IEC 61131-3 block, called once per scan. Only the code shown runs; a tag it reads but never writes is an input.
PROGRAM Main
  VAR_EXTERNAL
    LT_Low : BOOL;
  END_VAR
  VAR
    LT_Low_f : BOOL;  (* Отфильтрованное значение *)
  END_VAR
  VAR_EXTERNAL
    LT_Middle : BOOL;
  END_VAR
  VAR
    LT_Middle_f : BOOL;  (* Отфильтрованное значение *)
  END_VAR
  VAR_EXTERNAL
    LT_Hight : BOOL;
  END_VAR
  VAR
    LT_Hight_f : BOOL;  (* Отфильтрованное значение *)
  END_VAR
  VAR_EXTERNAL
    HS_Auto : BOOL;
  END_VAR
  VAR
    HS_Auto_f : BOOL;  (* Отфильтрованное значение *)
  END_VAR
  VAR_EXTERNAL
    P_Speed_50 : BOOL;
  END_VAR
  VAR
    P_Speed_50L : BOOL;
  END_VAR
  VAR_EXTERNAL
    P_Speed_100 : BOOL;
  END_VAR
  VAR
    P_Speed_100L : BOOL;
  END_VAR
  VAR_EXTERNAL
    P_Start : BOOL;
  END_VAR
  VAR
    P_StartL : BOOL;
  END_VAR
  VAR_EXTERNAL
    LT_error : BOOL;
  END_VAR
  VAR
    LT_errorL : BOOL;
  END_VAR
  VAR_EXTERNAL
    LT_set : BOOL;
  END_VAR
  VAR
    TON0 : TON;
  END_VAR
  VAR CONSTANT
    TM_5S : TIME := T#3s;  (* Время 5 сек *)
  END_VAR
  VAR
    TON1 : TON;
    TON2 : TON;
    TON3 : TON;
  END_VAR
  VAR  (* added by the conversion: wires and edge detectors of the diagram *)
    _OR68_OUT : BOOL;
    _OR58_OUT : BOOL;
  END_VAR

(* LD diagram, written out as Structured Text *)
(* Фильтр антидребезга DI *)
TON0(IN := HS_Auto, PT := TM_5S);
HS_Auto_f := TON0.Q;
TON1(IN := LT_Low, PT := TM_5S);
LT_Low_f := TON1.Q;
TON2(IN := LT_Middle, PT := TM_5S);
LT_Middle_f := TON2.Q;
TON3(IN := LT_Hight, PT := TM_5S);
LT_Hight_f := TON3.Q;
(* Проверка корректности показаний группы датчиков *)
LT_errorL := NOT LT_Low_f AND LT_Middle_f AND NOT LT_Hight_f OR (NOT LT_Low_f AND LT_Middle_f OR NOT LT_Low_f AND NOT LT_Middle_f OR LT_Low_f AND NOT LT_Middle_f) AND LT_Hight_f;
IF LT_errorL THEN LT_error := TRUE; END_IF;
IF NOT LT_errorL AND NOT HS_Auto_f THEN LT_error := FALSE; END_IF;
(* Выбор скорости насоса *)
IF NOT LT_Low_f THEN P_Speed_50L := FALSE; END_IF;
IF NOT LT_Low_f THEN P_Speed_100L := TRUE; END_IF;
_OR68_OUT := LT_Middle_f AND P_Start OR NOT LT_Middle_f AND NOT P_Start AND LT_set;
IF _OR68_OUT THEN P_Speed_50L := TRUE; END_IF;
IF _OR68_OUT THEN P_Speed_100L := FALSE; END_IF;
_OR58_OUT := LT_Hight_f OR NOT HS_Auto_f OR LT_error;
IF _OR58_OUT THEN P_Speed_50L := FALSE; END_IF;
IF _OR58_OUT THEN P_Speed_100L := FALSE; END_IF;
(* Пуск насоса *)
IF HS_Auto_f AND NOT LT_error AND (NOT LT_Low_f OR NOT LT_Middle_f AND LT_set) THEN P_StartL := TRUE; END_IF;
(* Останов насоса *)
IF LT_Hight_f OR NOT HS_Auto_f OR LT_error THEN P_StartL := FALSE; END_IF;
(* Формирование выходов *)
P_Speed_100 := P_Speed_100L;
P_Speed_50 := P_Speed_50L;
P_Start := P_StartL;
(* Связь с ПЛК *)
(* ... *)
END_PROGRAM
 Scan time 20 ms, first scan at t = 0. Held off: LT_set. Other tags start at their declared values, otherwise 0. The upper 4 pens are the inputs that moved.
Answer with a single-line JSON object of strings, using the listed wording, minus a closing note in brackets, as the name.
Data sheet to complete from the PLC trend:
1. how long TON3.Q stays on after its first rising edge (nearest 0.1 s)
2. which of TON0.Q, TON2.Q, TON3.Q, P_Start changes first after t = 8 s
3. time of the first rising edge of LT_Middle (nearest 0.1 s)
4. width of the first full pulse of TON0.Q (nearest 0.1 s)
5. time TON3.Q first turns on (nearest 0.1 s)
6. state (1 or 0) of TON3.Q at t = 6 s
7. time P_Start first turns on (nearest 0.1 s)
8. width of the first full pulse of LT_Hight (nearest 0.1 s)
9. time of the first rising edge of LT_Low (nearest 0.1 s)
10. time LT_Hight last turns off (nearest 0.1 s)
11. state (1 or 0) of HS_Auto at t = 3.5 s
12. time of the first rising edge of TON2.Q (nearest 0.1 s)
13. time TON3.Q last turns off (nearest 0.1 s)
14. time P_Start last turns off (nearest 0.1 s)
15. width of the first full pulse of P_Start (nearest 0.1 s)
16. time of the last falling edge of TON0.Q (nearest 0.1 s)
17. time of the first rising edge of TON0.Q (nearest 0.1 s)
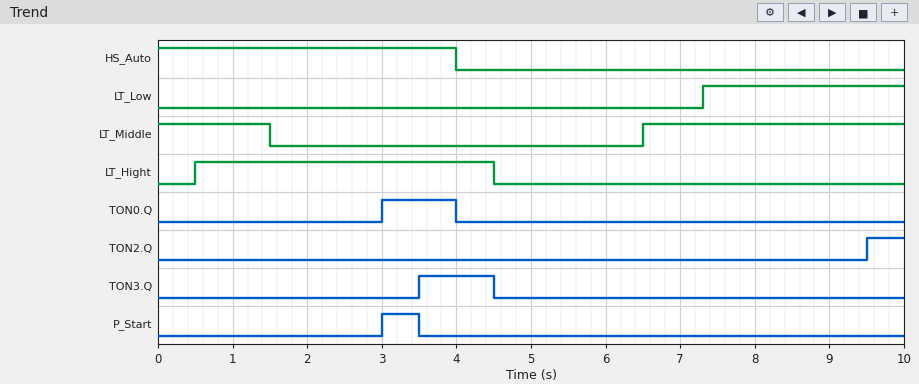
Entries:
{"how long TON3.Q stays on after its first rising edge": "1.0 s", "which of TON0.Q, TON2.Q, TON3.Q, P_Start changes first after t = 8 s": "TON2.Q", "time of the first rising edge of LT_Middle": "6.5 s", "width of the first full pulse of TON0.Q": "1.0 s", "time TON3.Q first turns on": "3.5 s", "state (1 or 0) of TON3.Q at t = 6 s": "0", "time P_Start first turns on": "3.0 s", "width of the first full pulse of LT_Hight": "4.0 s", "time of the first rising edge of LT_Low": "7.3 s", "time LT_Hight last turns off": "4.5 s", "state (1 or 0) of HS_Auto at t = 3.5 s": "1", "time of the first rising edge of TON2.Q": "9.5 s", "time TON3.Q last turns off": "4.5 s", "time P_Start last turns off": "3.5 s", "width of the first full pulse of P_Start": "0.5 s", "time of the last falling edge of TON0.Q": "4.0 s", "time of the first rising edge of TON0.Q": "3.0 s"}
